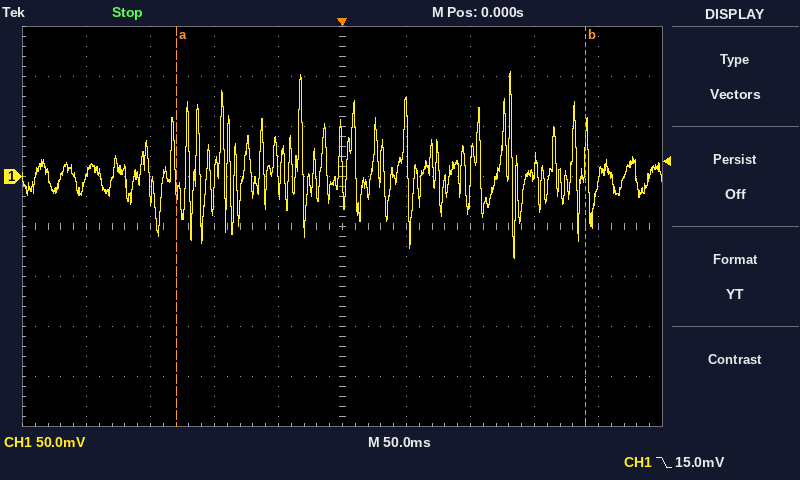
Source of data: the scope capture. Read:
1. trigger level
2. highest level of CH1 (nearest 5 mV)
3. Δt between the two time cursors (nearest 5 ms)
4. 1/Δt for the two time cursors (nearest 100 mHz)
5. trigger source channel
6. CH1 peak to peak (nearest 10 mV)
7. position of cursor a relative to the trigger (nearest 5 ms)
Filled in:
15.0 mV
105 mV
320 ms
3.1 Hz
CH1
190 mV
-130 ms
